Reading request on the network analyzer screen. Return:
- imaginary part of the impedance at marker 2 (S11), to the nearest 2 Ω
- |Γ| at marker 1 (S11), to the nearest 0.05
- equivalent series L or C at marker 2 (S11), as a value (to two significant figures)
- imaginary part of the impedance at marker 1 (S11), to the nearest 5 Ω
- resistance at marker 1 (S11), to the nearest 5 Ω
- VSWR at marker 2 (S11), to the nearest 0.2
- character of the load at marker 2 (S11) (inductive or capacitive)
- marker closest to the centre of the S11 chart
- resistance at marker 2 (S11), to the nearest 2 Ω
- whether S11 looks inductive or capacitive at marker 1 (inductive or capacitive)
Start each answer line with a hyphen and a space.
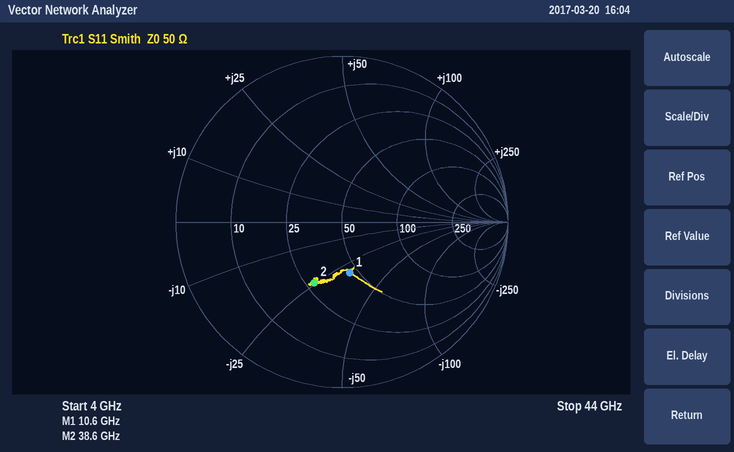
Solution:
- -24 Ω
- 0.30
- 170 fF
- -30 Ω
- 45 Ω
- 2.4
- capacitive
- marker 1
- 28 Ω
- capacitive
